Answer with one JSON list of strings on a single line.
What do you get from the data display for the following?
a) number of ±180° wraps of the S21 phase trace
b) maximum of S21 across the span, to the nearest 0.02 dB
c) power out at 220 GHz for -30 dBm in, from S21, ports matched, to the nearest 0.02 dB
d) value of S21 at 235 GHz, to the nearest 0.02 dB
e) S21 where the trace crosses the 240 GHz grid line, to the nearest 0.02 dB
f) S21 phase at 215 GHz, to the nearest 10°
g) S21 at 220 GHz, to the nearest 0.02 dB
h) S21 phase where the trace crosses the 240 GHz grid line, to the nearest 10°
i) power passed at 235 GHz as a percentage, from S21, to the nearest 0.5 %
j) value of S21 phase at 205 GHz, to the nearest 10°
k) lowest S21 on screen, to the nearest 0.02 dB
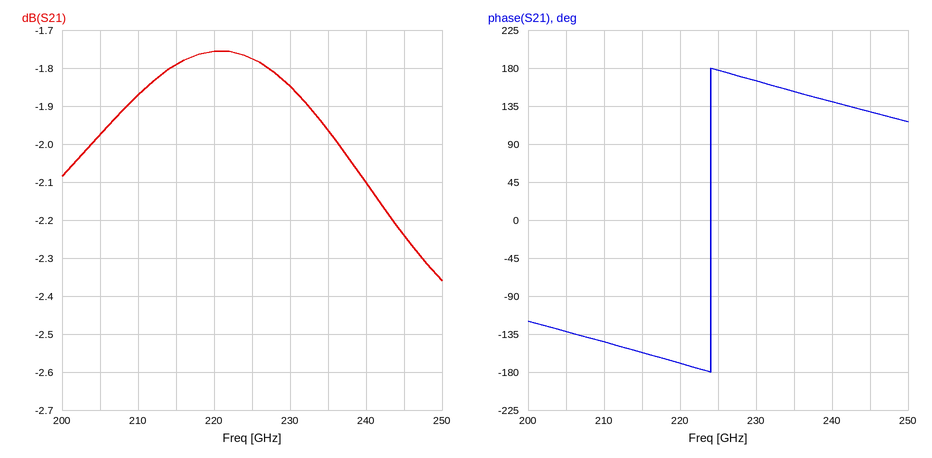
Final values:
["1", "-1.76 dB", "-31.76 dBm", "-1.96 dB", "-2.10 dB", "-160°", "-1.76 dB", "140°", "63.5 %", "-130°", "-2.36 dB"]
